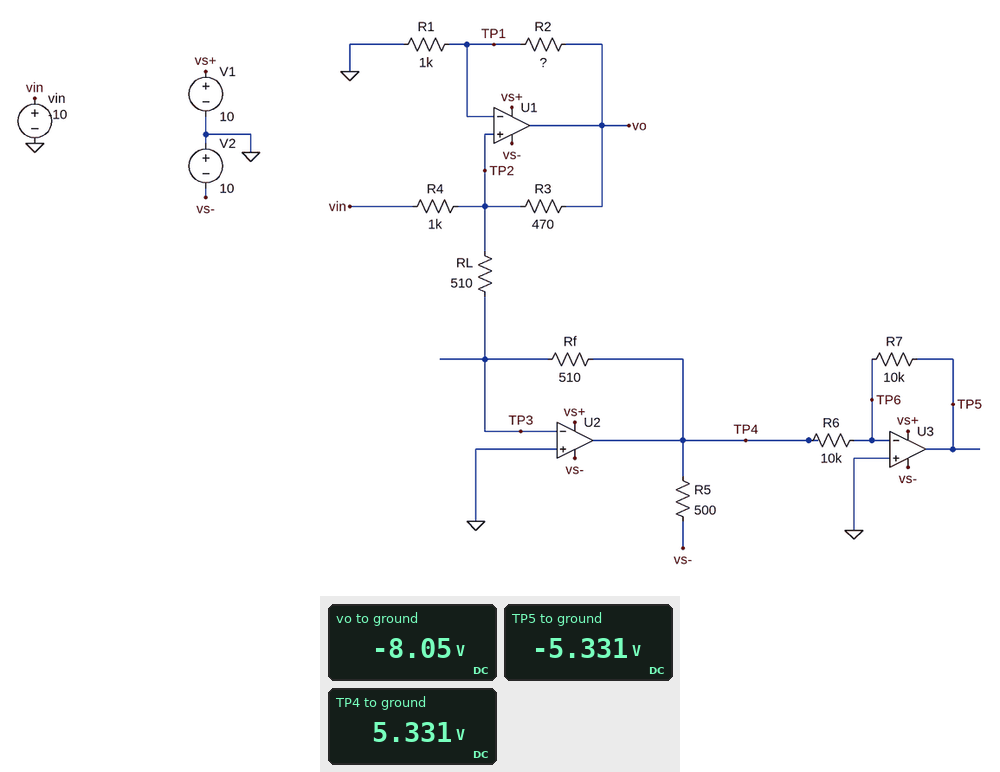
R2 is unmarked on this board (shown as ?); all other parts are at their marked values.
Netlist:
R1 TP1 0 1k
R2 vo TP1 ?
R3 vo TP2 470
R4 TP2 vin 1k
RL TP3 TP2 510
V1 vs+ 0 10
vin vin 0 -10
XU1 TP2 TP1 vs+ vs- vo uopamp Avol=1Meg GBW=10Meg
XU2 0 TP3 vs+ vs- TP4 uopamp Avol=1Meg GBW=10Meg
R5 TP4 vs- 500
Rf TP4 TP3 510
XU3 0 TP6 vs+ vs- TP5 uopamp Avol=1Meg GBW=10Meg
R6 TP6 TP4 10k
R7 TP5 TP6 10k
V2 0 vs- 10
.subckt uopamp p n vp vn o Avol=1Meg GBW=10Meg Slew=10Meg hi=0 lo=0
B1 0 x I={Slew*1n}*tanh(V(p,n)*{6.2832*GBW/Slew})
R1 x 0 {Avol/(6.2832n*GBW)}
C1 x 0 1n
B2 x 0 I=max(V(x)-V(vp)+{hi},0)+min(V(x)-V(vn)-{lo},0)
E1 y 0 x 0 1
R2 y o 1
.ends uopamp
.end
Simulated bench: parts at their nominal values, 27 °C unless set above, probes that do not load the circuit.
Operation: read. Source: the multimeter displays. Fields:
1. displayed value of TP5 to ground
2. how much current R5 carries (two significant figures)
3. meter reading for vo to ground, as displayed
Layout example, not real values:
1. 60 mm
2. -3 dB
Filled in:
1. -5.331 V
2. 31 mA
3. -8.05 V
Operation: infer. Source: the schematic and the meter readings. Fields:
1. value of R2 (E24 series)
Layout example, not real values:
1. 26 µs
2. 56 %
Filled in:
1. 510 Ω
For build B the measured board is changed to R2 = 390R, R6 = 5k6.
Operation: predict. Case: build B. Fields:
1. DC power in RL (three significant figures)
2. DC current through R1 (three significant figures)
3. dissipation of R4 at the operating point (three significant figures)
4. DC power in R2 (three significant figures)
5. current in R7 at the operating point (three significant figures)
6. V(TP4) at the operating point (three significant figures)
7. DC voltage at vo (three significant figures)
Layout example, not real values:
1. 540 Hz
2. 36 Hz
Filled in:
1. 43.2 mW
2. 4.69 mA
3. 28.2 mW
4. 8.59 mW
5. 838 µA
6. 4.69 V
7. -6.52 V
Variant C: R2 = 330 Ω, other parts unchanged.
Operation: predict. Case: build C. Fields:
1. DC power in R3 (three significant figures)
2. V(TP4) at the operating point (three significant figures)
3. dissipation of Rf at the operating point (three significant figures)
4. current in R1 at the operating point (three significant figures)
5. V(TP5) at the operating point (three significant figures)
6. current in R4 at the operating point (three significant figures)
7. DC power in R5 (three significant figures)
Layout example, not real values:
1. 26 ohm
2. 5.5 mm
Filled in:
1. 4.54 mW
2. 4.43 V
3. 38.4 mW
4. 4.43 mA
5. -4.43 V
6. 5.57 mA
7. 416 mW
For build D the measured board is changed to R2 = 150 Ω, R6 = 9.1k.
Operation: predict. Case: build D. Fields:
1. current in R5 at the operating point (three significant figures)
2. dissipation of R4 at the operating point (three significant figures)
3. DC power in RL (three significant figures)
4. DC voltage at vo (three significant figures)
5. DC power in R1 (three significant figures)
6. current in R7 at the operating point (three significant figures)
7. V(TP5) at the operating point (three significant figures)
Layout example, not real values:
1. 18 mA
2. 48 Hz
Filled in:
1. 27.6 mA
2. 38.6 mW
3. 28.1 mW
4. -4.35 V
5. 14.3 mW
6. 416 µA
7. -4.16 V
